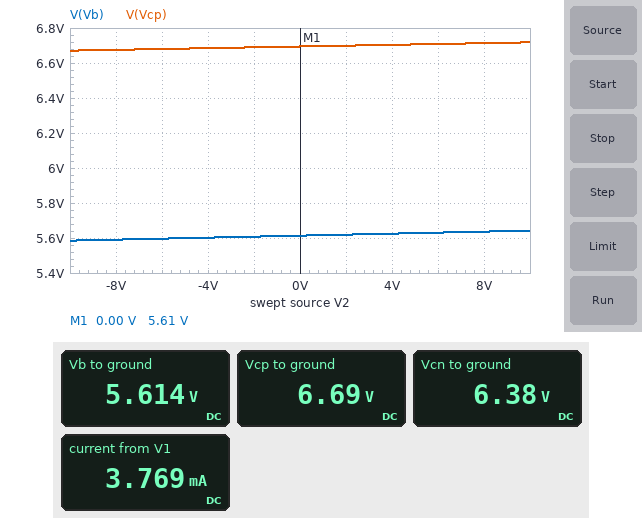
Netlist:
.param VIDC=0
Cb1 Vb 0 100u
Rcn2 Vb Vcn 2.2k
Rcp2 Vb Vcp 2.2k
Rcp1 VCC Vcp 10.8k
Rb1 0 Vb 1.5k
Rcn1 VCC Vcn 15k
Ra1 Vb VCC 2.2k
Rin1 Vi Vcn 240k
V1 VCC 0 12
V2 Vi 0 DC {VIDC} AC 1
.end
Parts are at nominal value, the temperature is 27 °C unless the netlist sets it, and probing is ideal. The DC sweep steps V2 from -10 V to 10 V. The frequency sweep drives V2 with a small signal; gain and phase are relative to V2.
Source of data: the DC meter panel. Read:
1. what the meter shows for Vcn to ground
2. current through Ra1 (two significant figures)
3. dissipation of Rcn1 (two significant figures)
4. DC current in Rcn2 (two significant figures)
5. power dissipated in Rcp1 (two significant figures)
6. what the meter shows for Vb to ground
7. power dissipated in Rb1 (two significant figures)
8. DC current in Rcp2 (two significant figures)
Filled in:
6.38 V
2.9 mA
2.1 mW
350 µA
2.6 mW
5.614 V
21 mW
490 µA
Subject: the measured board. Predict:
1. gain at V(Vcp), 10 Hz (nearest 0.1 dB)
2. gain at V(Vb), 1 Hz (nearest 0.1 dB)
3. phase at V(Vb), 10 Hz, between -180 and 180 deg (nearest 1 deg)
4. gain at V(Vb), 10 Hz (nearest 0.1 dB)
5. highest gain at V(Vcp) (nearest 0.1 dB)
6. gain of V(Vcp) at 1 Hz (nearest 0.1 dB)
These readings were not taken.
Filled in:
-66.6 dB
-51.8 dB
-79 deg
-65.0 dB
-52.5 dB
-53.4 dB
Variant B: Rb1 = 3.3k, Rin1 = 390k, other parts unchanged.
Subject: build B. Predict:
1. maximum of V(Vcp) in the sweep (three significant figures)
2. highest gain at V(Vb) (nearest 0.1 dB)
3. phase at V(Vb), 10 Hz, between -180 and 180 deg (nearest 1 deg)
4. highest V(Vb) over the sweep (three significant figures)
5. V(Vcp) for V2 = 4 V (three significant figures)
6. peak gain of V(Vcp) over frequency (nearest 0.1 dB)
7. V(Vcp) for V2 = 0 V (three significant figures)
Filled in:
8.62 V
-52.1 dB
-82 deg
7.93 V
8.61 V
-53.7 dB
8.60 V
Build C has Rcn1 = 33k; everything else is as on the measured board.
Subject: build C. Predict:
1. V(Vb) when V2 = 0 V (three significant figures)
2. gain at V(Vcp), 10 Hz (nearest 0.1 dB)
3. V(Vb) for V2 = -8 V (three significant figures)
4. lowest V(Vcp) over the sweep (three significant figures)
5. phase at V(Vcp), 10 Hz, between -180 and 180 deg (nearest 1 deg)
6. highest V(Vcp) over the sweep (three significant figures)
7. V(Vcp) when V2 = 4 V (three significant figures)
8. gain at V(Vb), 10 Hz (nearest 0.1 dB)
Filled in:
5.46 V
-66.0 dB
5.43 V
6.54 V
-79 deg
6.59 V
6.58 V
-64.4 dB
